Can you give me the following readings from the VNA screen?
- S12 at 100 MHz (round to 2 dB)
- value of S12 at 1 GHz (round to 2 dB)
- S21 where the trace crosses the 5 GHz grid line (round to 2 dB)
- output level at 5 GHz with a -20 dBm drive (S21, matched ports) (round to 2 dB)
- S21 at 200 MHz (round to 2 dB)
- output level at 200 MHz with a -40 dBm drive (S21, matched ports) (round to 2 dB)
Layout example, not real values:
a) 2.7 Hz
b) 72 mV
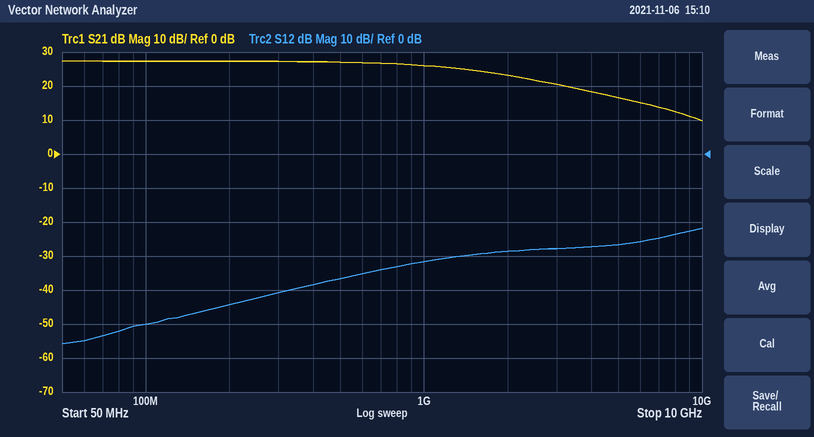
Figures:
a) -50 dB
b) -32 dB
c) 16 dB
d) -4 dBm
e) 28 dB
f) -12 dBm
